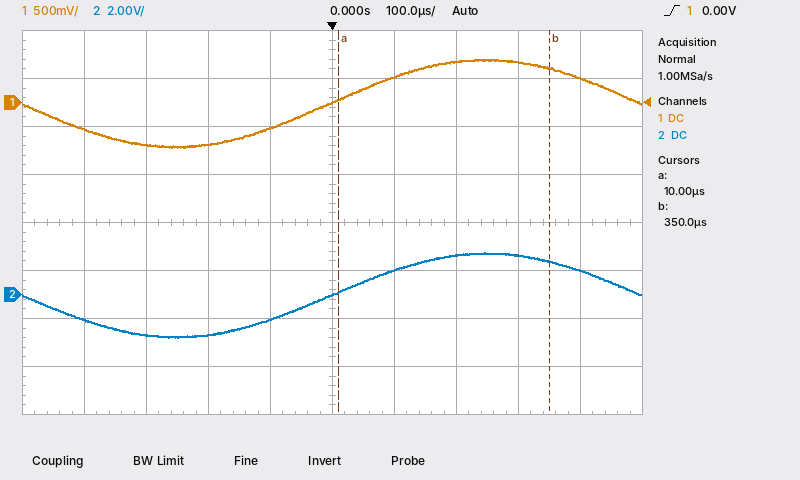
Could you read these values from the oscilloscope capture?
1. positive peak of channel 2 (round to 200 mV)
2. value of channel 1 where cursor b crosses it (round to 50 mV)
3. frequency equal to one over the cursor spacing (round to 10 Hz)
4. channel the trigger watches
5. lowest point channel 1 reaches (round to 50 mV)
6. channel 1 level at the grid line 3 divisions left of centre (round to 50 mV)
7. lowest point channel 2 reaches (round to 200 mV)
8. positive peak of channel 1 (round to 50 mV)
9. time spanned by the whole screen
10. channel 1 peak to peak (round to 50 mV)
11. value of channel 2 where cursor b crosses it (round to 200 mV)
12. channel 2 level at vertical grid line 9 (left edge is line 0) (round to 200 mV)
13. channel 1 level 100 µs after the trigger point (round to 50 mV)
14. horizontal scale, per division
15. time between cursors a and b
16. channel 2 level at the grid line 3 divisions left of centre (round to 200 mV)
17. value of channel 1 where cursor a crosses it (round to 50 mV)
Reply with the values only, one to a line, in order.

1.8 V
350 mV
2.94 kHz
channel 1
-450 mV
-450 mV
-1.8 V
450 mV
1 ms
900 mV
1.4 V
1.0 V
250 mV
100 µs
340 µs
-1.6 V
50 mV
